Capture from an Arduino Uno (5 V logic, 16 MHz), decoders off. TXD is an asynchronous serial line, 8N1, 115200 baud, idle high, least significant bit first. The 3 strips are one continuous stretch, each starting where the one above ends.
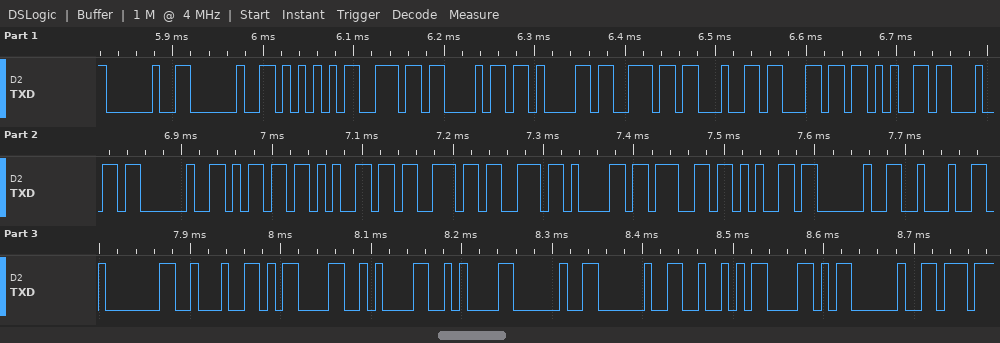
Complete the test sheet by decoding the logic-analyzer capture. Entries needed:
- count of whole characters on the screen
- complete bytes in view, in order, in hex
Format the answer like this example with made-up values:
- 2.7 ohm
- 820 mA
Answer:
- 31
- 20 20 55 6E 68 61 6E 64 6C 65 64 20 6D 65 73 73 61 67 65 20 22 01 22 0D 0A 0A 20 20 52 58 20
